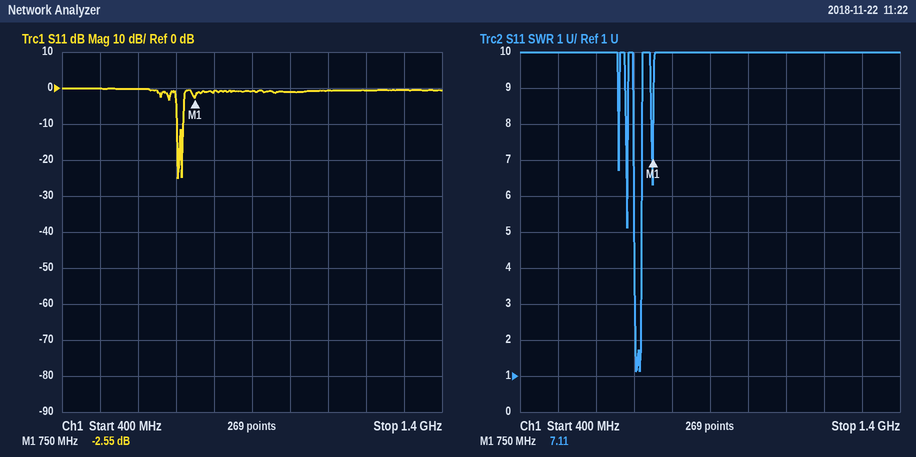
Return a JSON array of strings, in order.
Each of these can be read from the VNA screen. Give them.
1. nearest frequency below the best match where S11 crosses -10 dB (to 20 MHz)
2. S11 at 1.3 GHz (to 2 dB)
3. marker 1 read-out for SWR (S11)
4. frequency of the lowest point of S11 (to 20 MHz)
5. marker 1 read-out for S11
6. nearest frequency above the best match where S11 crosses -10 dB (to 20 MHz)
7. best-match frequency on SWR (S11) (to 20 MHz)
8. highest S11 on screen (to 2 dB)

["700 MHz", "0 dB", "7.11", "700 MHz", "-2.55 dB", "720 MHz", "700 MHz", "0 dB"]
